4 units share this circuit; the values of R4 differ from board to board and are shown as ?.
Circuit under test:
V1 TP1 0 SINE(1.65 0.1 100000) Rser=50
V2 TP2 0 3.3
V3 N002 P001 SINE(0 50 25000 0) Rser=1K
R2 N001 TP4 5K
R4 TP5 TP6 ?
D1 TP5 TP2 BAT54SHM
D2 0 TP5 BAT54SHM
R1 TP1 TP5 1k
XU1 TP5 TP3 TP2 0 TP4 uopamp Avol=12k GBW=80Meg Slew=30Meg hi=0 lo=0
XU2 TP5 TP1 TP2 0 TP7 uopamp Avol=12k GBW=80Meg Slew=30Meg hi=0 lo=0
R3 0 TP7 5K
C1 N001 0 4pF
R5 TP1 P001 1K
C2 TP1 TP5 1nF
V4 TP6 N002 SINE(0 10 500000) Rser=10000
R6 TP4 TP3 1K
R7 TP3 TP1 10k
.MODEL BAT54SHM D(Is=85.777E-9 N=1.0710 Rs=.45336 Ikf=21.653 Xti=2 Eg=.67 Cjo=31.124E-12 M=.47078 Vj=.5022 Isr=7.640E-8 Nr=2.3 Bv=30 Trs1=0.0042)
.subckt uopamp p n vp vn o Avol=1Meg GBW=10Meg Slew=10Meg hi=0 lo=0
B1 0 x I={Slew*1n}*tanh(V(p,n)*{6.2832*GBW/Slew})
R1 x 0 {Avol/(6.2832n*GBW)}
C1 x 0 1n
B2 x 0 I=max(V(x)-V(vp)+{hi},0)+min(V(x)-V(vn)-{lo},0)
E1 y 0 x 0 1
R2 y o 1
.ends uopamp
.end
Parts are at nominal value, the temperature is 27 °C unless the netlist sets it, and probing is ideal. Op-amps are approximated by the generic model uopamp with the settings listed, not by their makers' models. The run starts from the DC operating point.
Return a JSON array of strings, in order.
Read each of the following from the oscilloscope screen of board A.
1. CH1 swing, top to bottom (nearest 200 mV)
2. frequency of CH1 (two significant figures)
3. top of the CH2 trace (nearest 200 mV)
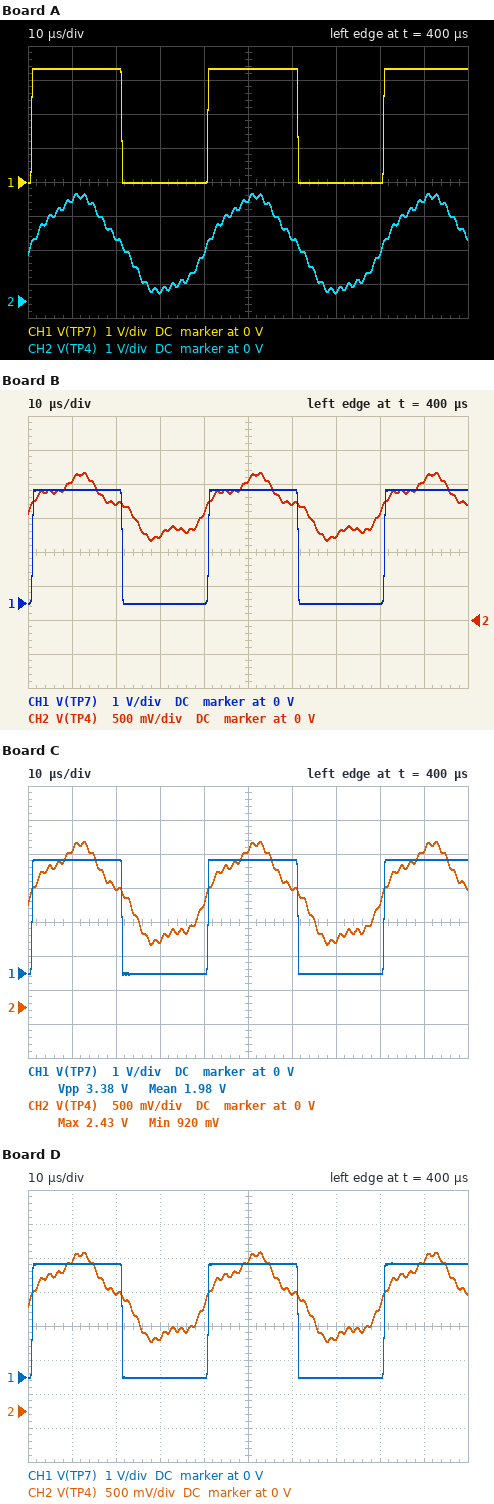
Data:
["3.4 V", "25 kHz", "3.2 V"]
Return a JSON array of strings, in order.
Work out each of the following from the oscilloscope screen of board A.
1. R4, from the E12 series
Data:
["27 kΩ"]
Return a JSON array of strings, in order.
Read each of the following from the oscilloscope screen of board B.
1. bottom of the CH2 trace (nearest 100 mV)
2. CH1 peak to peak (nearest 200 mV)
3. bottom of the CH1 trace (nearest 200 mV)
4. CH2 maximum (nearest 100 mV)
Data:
["1.2 V", "3.4 V", "0 V", "2.2 V"]
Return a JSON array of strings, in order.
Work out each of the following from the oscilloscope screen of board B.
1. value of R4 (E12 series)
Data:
["120 kΩ"]
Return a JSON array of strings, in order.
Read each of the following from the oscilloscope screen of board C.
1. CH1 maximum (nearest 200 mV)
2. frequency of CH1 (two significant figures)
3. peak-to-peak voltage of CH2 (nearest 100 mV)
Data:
["3.4 V", "25 kHz", "1.5 V"]
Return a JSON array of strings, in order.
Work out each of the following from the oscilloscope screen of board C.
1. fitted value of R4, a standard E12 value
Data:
["68 kΩ"]
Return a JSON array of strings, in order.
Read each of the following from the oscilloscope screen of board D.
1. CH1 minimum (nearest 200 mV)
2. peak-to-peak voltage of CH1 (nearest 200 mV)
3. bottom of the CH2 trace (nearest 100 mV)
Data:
["0 V", "3.4 V", "1.0 V"]
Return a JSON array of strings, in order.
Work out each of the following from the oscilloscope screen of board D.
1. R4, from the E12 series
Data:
["82 kΩ"]
